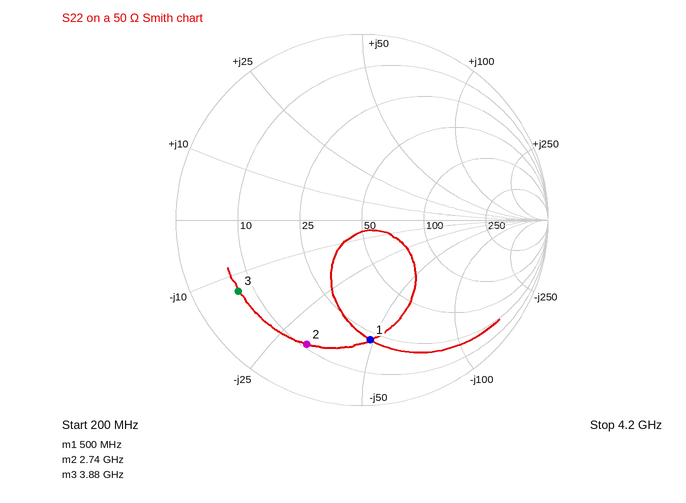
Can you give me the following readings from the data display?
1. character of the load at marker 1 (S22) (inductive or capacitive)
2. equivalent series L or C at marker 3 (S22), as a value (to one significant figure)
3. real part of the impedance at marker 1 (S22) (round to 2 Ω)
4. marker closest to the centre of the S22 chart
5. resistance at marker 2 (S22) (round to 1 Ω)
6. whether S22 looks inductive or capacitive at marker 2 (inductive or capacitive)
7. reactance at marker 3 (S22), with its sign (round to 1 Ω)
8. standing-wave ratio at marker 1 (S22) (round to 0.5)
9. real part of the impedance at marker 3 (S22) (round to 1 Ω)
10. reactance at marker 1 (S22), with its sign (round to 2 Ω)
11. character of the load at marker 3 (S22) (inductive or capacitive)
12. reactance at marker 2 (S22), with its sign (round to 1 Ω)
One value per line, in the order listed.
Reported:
capacitive
3 pF
22 Ω
marker 1
11 Ω
capacitive
-13 Ω
4.5
7 Ω
-48 Ω
capacitive
-31 Ω
